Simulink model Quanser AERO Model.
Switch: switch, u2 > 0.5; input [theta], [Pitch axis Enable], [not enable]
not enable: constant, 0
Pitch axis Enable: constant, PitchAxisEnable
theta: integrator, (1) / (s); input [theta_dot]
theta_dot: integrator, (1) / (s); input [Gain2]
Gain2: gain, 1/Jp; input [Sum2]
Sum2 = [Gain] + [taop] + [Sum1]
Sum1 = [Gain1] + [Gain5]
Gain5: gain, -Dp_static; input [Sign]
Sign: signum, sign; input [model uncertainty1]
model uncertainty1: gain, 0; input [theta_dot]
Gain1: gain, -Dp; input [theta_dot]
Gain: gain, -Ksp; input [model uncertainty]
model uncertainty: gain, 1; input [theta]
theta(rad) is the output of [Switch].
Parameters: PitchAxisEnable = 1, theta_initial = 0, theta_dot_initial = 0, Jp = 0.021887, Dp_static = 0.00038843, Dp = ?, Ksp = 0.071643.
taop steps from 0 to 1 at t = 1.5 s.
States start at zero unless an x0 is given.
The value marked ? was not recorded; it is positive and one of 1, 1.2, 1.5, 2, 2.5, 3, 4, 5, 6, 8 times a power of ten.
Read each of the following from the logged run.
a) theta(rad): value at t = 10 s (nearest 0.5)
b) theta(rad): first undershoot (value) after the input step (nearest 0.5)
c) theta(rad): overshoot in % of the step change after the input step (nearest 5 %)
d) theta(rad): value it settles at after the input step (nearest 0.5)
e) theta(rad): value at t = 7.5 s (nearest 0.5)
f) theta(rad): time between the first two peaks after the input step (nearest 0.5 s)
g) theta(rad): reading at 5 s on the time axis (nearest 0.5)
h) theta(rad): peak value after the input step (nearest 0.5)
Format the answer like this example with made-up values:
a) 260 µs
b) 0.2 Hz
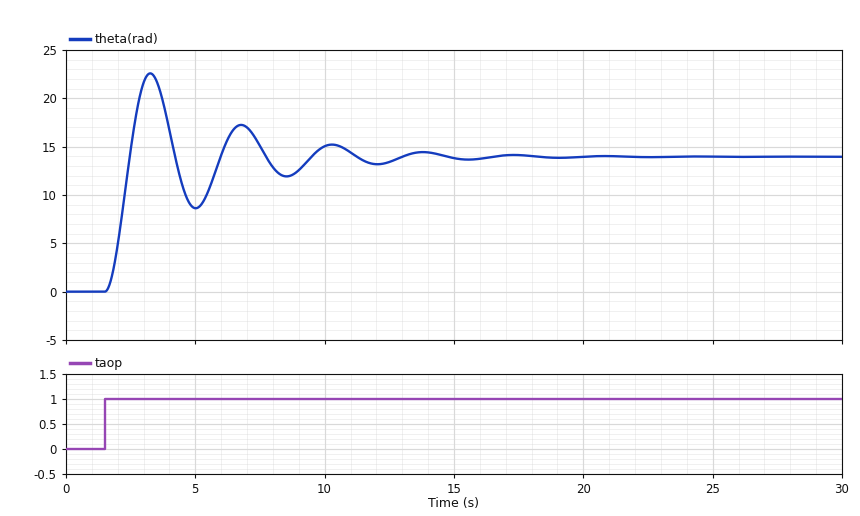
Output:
a) 15.0
b) 8.5
c) 60 %
d) 14.0
e) 15.0
f) 3.5 s
g) 8.5
h) 22.5
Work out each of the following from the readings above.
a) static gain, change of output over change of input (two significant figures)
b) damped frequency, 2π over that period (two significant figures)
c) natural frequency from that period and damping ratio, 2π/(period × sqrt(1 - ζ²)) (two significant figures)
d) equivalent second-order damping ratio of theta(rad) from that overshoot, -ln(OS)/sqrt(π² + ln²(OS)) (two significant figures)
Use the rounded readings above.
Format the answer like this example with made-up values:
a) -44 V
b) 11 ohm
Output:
a) 14
b) 1.8 rad/s
c) 1.8 rad/s
d) 0.16
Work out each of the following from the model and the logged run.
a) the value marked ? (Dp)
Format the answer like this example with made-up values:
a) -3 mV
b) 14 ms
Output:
a) 0.012
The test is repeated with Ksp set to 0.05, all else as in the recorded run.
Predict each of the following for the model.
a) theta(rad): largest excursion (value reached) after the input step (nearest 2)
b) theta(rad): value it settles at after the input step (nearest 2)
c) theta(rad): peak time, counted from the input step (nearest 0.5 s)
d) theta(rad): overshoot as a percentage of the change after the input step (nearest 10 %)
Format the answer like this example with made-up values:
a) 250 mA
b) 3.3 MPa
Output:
a) 32
b) 20
c) 2.0 s
d) 60 %
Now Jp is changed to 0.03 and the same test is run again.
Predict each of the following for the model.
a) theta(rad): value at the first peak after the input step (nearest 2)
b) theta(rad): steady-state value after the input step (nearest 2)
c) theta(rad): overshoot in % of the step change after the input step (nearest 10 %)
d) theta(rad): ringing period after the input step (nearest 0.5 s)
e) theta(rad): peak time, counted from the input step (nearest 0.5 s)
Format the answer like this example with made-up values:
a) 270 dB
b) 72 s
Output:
a) 24
b) 14
c) 70 %
d) 4.0 s
e) 2.0 s
